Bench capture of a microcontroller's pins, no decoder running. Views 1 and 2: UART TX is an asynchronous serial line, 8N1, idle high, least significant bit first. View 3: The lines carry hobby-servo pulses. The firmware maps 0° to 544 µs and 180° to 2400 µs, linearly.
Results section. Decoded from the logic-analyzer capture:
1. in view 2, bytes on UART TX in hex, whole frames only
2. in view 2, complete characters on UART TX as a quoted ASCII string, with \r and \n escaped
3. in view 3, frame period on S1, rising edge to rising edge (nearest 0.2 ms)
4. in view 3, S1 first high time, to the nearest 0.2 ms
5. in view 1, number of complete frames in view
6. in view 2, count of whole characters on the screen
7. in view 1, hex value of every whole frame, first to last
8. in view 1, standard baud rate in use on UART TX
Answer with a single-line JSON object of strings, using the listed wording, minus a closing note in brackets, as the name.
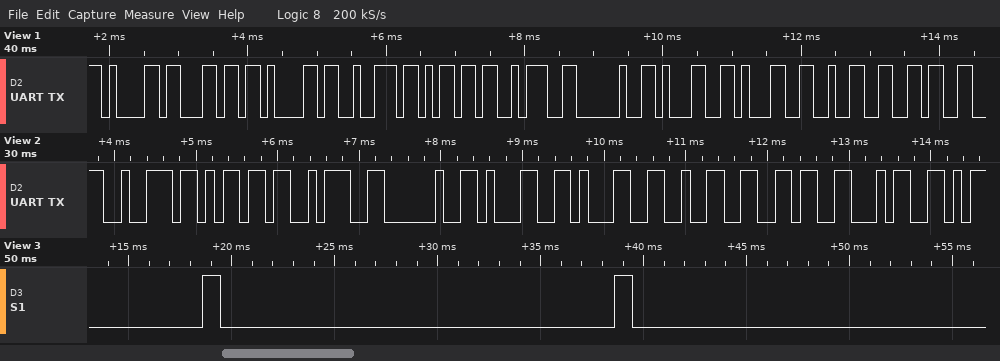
{"in view 2, bytes on UART TX in hex, whole frames only": "0x72 0x6D 0x3A 0x20 0x31 0x31 0x32 0x36 0x34", "in view 2, complete characters on UART TX as a quoted ASCII string, with \\r and \\n escaped": "\"rm: 11264\"", "in view 3, frame period on S1, rising edge to rising edge": "20.0 ms", "in view 3, S1 first high time, to the nearest 0.2 ms": "0.8 ms", "in view 1, number of complete frames in view": "11", "in view 2, count of whole characters on the screen": "9", "in view 1, hex value of every whole frame, first to last": "0x61 0x6C 0x61 0x72 0x6D 0x3A 0x20 0x31 0x31 0x32 0x36", "in view 1, standard baud rate in use on UART TX": "9600 baud"}
